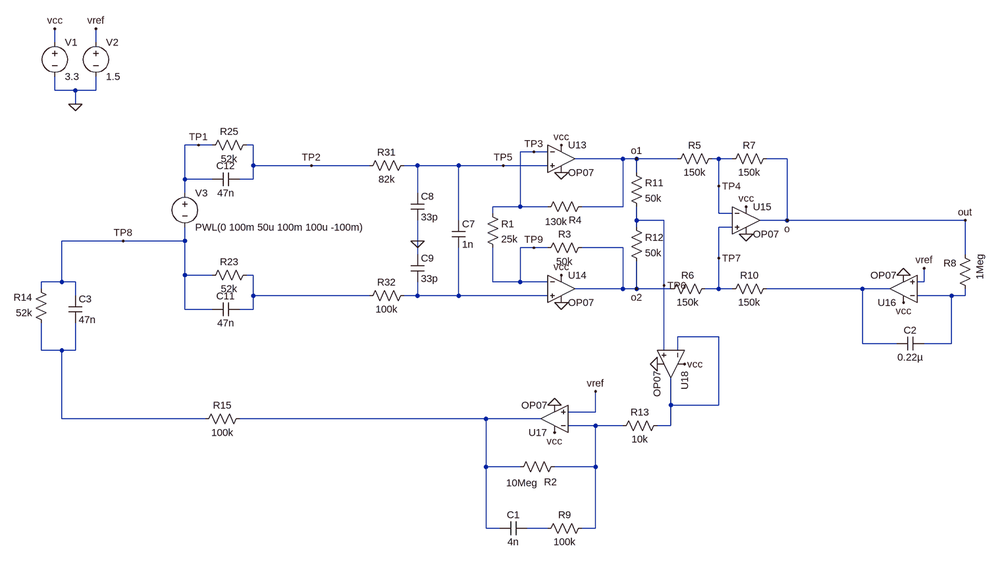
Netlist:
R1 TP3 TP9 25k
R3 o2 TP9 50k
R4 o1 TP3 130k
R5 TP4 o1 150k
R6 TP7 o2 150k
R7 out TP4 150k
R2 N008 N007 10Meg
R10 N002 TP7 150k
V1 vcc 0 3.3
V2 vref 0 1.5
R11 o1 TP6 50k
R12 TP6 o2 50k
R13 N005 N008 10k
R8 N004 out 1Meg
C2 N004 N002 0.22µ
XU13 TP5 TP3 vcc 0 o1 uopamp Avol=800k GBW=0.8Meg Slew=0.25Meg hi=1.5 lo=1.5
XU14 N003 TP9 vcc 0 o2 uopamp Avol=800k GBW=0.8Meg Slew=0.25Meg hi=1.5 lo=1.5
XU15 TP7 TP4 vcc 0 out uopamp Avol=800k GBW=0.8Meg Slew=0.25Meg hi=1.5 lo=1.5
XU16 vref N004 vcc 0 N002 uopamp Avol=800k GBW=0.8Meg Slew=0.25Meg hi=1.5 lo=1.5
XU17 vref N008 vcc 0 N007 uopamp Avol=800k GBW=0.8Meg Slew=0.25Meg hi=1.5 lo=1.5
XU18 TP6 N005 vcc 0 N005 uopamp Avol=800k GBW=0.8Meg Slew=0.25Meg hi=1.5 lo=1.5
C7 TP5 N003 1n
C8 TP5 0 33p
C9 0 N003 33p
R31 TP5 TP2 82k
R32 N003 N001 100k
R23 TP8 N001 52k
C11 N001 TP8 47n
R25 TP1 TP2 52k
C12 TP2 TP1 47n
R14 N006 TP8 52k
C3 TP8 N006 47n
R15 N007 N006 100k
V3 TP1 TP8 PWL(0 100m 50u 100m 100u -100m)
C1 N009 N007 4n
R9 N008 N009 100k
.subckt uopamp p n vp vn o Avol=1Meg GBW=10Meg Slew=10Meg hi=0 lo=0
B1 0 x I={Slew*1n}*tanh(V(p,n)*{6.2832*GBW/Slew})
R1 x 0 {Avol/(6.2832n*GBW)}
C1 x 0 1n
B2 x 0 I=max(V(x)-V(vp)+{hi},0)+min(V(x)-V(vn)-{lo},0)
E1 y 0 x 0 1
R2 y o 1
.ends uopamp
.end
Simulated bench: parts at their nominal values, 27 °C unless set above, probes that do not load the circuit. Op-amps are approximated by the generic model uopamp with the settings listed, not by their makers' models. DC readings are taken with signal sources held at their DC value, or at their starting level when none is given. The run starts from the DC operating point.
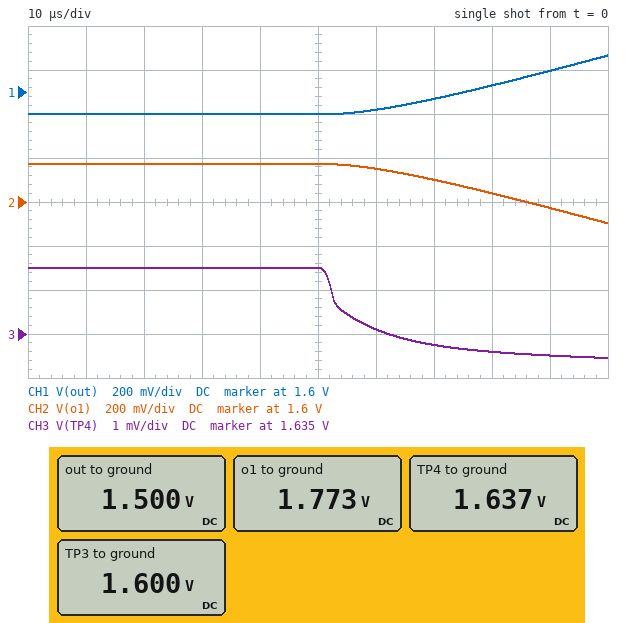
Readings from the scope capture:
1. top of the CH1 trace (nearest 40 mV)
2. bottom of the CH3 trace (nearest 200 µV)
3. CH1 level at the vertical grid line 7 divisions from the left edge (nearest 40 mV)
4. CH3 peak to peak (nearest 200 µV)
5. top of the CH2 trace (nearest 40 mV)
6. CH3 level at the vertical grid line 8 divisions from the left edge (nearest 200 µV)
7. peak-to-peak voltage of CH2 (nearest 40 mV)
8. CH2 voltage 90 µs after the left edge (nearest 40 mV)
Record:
1.76 V
1.6344 V
1.56 V
2.0 mV
1.76 V
1.6346 V
280 mV
1.56 V
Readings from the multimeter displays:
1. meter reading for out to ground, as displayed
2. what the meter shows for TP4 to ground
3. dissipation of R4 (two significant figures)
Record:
1.500 V
1.637 V
230 nW
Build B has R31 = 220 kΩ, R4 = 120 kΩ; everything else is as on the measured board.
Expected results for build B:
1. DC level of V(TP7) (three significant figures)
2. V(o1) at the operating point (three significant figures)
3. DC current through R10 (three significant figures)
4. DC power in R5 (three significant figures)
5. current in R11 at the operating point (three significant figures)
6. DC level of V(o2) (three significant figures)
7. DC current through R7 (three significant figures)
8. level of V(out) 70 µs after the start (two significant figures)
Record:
1.63 V
1.76 V
863 nA
112 nW
2.60 µA
1.50 V
866 nA
1.5 V
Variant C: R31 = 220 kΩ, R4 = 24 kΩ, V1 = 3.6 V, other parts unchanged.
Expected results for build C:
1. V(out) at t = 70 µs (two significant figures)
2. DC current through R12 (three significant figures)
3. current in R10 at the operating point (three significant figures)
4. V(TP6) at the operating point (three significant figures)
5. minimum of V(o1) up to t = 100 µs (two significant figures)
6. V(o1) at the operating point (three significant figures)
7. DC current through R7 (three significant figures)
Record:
1.5 V
1.32 µA
437 nA
1.57 V
1.6 V
1.63 V
439 nA
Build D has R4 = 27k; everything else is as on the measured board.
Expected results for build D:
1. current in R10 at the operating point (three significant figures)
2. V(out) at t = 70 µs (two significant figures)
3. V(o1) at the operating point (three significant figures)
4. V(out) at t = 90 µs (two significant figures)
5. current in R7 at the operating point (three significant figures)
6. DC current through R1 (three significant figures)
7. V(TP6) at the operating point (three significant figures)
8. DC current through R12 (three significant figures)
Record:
451 nA
1.5 V
1.64 V
1.6 V
453 nA
1.33 µA
1.57 V
1.36 µA
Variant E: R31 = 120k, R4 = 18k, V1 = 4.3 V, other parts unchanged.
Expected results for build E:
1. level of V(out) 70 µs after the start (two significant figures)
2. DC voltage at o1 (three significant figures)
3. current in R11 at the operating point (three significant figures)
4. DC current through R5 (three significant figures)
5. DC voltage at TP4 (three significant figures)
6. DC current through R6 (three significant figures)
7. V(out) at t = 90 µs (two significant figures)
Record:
1.5 V
1.62 V
1.24 µA
413 nA
1.56 V
411 nA
1.6 V
